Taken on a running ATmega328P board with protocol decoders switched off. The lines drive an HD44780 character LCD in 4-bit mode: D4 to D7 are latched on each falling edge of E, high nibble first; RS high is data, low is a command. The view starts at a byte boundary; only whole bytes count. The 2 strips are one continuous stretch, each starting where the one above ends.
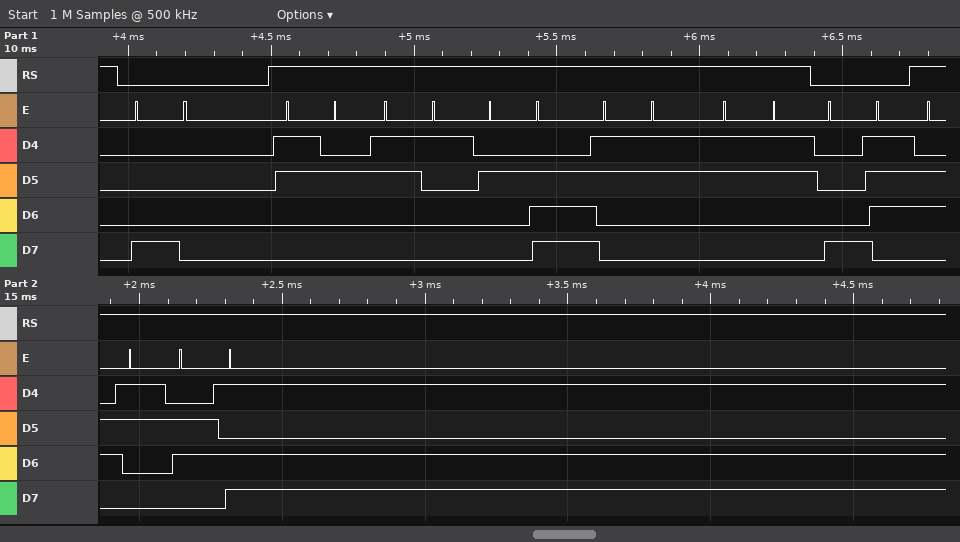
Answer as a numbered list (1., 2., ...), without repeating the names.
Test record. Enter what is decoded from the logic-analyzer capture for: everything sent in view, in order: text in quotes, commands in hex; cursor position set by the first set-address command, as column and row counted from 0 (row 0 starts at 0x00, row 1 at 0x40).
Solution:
1. 0x80 "21.33" 0x87 "cm"
2. column 0, row 0
